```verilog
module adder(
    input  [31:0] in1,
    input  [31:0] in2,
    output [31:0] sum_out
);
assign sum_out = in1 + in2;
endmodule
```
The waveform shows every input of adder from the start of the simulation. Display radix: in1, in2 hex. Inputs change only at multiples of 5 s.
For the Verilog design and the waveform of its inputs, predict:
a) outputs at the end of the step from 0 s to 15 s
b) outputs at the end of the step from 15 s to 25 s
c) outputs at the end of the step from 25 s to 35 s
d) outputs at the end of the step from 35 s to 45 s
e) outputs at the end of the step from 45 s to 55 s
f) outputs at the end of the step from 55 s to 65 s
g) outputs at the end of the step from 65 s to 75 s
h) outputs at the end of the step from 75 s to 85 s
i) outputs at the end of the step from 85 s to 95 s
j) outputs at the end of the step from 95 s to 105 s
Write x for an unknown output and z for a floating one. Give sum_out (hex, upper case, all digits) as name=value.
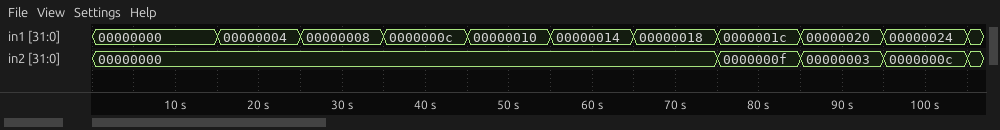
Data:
sum_out=00000000
sum_out=00000004
sum_out=00000008
sum_out=0000000C
sum_out=00000010
sum_out=00000014
sum_out=00000018
sum_out=0000002B
sum_out=00000023
sum_out=00000030
